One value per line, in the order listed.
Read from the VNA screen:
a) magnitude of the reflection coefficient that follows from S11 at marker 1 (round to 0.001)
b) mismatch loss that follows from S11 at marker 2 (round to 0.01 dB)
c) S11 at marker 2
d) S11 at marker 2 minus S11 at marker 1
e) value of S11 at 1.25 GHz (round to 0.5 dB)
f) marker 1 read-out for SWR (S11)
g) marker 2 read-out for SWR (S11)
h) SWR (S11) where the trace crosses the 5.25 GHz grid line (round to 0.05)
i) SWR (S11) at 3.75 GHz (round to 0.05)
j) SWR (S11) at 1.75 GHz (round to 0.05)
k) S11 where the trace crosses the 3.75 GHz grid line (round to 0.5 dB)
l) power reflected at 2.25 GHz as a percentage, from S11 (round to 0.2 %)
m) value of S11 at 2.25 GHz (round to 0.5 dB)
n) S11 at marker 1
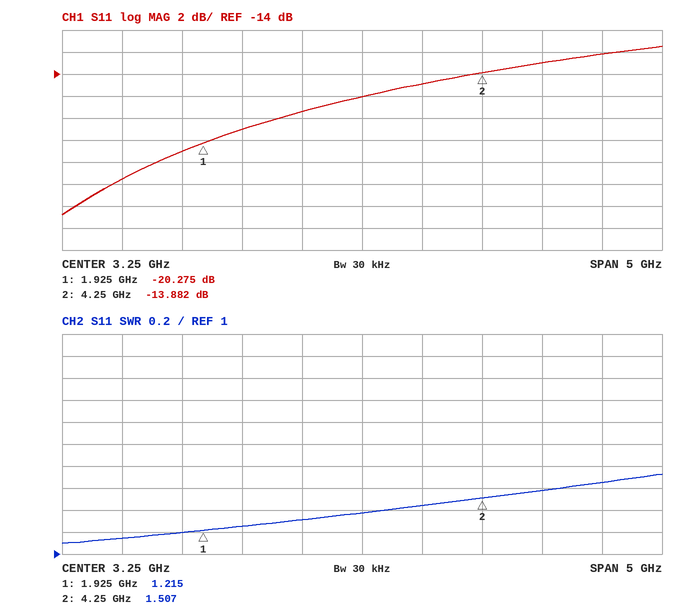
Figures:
0.097
0.18 dB
-13.882 dB
6.393 dB
-23.5 dB
1.215
1.507
1.65
1.45
1.20
-15.0 dB
1.2 %
-19.0 dB
-20.275 dB
